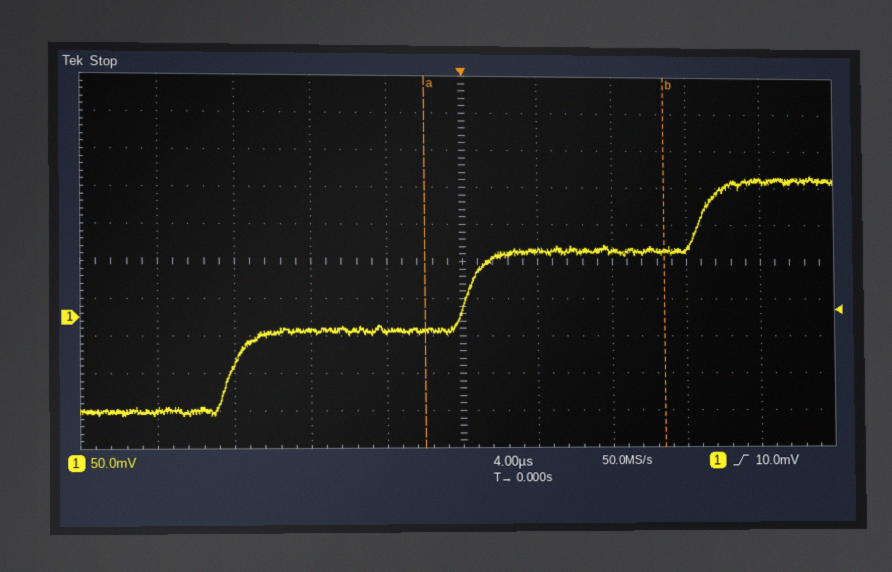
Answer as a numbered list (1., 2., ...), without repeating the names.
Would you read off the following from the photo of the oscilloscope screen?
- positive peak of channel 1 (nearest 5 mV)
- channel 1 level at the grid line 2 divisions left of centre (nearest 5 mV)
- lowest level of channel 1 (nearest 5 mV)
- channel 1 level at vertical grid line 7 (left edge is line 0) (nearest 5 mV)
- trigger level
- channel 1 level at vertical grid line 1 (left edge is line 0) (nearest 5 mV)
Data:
1. 190 mV
2. -15 mV
3. -130 mV
4. 90 mV
5. 10.0 mV
6. -125 mV
